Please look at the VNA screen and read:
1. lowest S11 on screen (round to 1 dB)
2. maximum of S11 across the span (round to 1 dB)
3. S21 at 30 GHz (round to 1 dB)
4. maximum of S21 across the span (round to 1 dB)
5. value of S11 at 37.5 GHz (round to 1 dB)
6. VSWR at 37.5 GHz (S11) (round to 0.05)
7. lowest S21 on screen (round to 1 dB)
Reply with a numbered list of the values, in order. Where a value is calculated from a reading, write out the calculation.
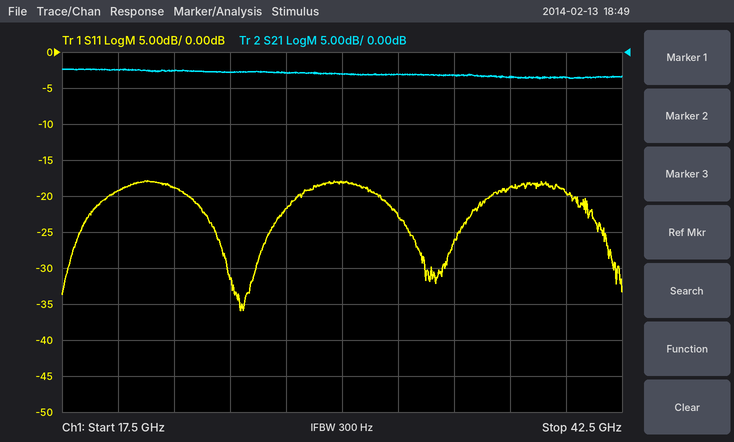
1. -36 dB
2. -18 dB
3. -3 dB
4. -2 dB
5. -19 dB
6. |Γ| = 10^(-19/20) = 0.1122; VSWR = (1 + 0.1122)/(1 − 0.1122) ≈ 1.25
7. -4 dB
